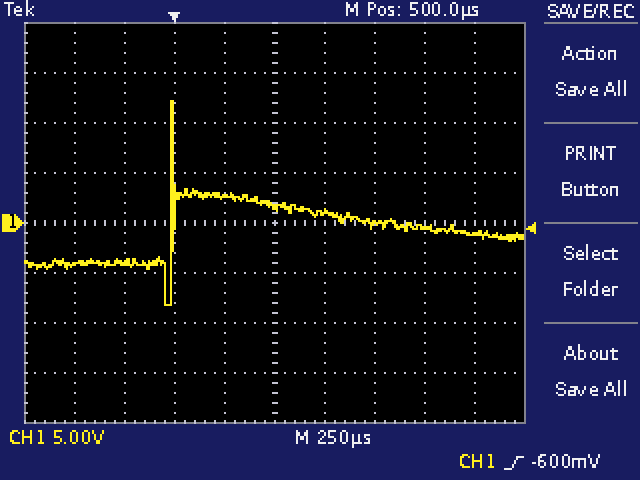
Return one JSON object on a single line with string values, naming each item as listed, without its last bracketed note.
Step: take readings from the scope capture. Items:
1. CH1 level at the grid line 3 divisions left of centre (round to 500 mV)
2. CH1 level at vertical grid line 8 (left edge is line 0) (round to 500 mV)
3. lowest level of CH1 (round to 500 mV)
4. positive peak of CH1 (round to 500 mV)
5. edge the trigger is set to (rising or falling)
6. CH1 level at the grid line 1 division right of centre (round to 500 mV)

{"CH1 level at the grid line 3 divisions left of centre": "-4.0 V", "CH1 level at vertical grid line 8 (left edge is line 0)": "-500 mV", "lowest level of CH1": "-8.0 V", "positive peak of CH1": "12.0 V", "edge the trigger is set to": "rising", "CH1 level at the grid line 1 division right of centre": "1.0 V"}
